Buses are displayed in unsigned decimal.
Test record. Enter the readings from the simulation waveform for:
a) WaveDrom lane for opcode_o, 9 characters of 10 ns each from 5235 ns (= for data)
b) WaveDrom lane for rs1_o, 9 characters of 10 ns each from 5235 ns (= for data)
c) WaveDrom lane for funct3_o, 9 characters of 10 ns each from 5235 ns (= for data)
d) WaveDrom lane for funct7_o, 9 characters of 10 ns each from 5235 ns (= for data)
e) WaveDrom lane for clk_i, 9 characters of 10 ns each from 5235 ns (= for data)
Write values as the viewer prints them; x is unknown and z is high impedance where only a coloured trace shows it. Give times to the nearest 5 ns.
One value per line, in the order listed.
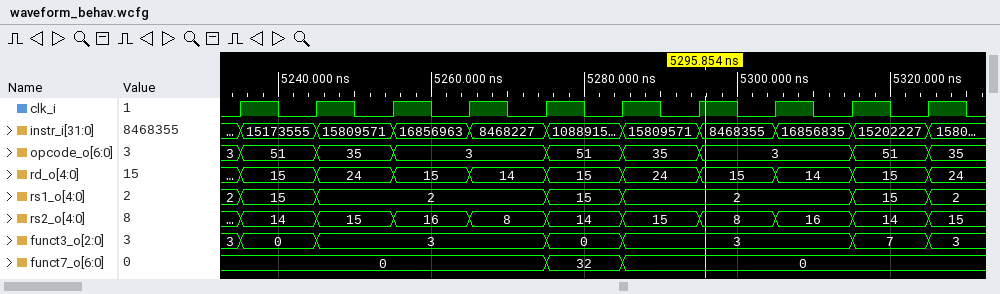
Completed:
{name: 'opcode_o', wave: '===.===.=', data: '51 35 3 51 35 3 51'}
{name: 'rs1_o', wave: '==..==..=', data: '15 2 15 2 15'}
{name: 'funct3_o', wave: '==..==..=', data: '0 3 0 3 7'}
{name: 'funct7_o', wave: '=...==...', data: '0 32 0'}
{name: 'clk_i', wave: 'p........'}
